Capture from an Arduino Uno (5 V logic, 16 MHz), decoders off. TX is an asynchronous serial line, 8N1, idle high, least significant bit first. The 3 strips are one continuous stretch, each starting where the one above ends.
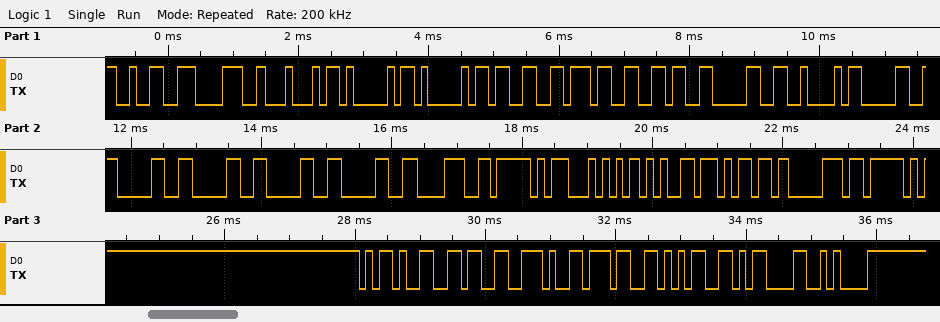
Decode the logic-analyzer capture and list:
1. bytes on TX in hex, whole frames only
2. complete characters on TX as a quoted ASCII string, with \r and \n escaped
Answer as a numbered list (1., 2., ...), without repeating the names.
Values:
1. 32 38 44 41 41 33 37 36 30 42 30 30 30 30 30 38 5F 54 65 6D 70 5F 2D 36 2E 37 35 0D 0A
2. "28DAA3760B000008_Temp_-6.75\r\n"
